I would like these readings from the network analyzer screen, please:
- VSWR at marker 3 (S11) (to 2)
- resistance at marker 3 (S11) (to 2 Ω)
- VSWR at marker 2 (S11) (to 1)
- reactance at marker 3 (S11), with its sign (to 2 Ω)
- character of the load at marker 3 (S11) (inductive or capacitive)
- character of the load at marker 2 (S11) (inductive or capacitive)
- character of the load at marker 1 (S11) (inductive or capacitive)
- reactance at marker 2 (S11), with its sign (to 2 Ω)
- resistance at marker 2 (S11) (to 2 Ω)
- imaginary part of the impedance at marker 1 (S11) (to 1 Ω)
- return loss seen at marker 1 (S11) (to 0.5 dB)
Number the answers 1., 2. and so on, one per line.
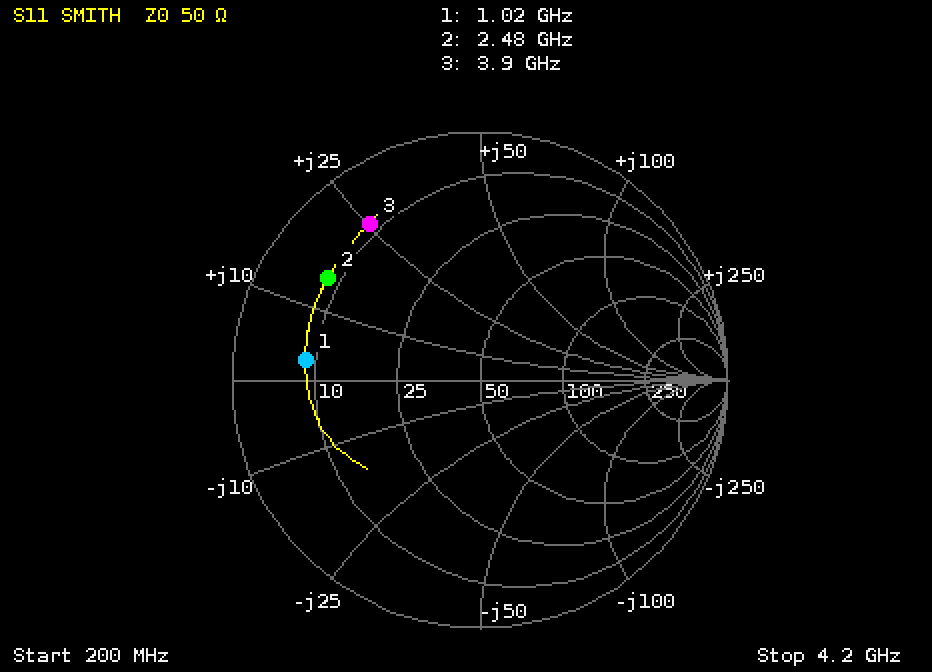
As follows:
1. 8
2. 8 Ω
3. 7
4. +26 Ω
5. inductive
6. inductive
7. inductive
8. +14 Ω
9. 8 Ω
10. +3 Ω
11. 3.0 dB
